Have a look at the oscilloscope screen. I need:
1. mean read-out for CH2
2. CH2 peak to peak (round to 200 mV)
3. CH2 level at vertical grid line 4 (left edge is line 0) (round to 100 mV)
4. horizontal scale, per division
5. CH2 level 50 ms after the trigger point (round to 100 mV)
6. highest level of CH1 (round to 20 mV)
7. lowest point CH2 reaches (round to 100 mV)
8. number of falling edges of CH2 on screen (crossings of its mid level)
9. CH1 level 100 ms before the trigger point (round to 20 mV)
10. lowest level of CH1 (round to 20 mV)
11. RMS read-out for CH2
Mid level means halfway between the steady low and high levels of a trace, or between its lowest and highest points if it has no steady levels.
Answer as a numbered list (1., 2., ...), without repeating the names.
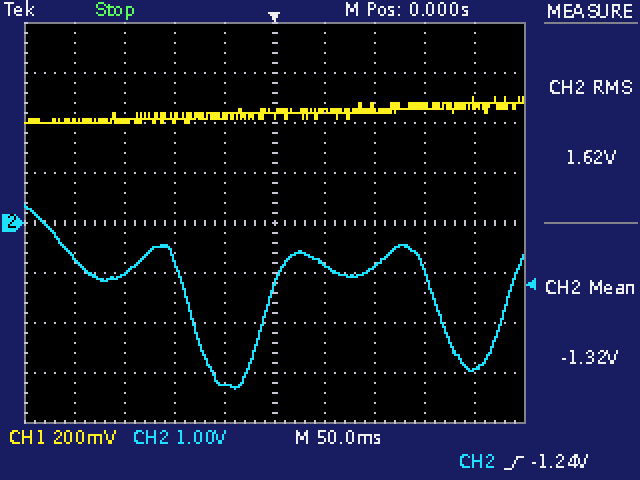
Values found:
1. -1.32 V
2. 3.6 V
3. -3.2 V
4. 50 ms
5. -800 mV
6. 500 mV
7. -3.3 V
8. 2
9. 420 mV
10. 400 mV
11. 1.62 V
